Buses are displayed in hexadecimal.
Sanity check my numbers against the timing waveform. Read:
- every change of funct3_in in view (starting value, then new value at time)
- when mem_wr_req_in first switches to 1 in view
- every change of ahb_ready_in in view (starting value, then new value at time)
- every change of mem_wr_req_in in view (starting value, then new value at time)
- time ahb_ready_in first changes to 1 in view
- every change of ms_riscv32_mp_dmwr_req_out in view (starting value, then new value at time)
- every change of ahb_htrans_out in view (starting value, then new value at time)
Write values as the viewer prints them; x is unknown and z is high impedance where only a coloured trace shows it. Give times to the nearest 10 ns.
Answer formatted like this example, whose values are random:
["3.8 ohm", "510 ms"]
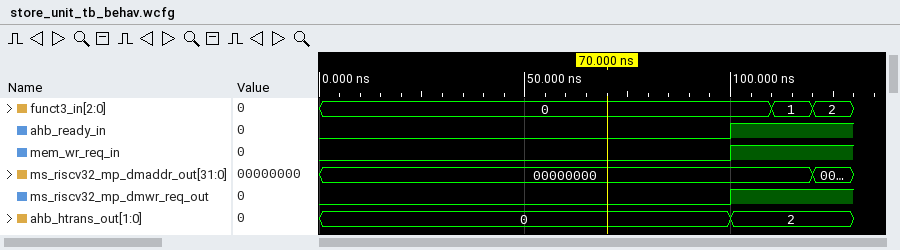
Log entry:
["0, 1 at 110 ns, 2 at 120 ns", "100 ns", "0, 1 at 100 ns", "0, 1 at 100 ns", "100 ns", "0, 1 at 100 ns", "0, 2 at 100 ns"]
